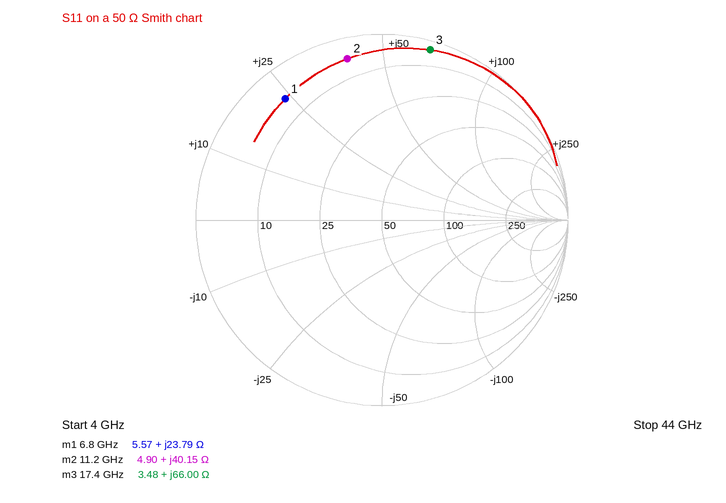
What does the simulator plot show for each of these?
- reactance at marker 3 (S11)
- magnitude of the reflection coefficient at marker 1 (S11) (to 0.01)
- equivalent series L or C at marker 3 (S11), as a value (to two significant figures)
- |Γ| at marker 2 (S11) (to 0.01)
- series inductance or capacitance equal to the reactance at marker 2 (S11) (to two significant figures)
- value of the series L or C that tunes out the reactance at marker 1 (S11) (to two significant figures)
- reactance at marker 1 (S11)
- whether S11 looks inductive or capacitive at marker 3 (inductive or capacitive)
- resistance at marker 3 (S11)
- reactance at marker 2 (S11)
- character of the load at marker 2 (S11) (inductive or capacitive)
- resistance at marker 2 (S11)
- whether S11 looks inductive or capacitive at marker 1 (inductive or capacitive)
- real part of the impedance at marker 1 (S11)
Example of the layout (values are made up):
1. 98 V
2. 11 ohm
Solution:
1. +66.00 Ω
2. 0.83
3. 600 pH
4. 0.89
5. 570 pH
6. 980 fF
7. +23.79 Ω
8. inductive
9. 3.48 Ω
10. +40.15 Ω
11. inductive
12. 4.90 Ω
13. inductive
14. 5.57 Ω
